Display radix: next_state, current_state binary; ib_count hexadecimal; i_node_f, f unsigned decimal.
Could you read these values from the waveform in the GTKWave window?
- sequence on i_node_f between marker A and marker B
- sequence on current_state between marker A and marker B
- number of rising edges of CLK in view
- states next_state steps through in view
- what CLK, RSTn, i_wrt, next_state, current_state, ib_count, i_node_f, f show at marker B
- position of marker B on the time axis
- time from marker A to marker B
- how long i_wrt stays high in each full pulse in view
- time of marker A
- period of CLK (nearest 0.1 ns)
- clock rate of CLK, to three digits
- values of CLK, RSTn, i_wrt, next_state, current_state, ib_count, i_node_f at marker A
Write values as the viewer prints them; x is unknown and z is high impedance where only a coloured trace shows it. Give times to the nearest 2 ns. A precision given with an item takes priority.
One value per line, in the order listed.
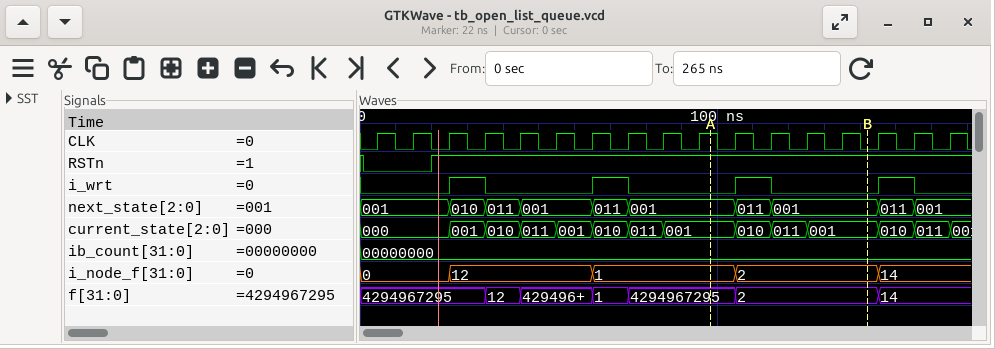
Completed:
1, 2
001, 010, 011, 001
17
001, 010, 011, 001, 011, 001, 011, 001, 011, 001
CLK=0, RSTn=1, i_wrt=0, next_state=001, current_state=001, ib_count=00000000, i_node_f=2, f=2
142 ns
44 ns
10 ns, 10 ns, 10 ns, 10 ns
98 ns
10 ns
100 MHz
CLK=1, RSTn=1, i_wrt=0, next_state=001, current_state=001, ib_count=00000000, i_node_f=1
